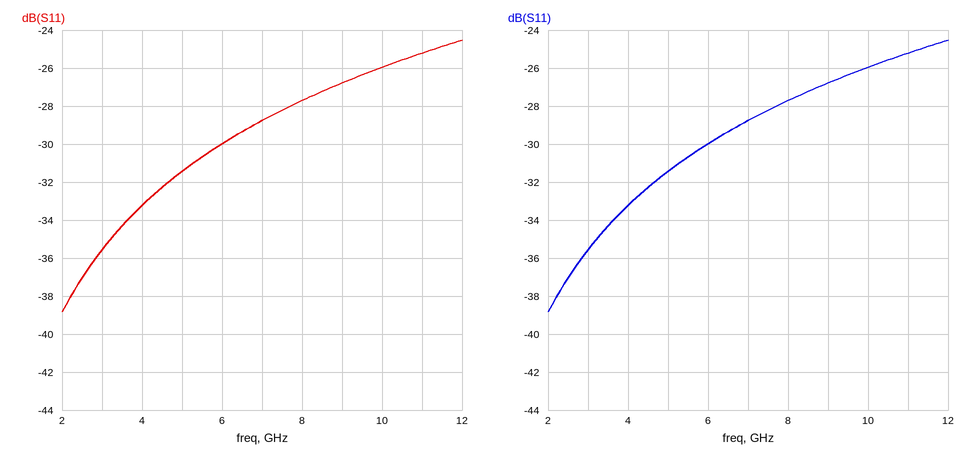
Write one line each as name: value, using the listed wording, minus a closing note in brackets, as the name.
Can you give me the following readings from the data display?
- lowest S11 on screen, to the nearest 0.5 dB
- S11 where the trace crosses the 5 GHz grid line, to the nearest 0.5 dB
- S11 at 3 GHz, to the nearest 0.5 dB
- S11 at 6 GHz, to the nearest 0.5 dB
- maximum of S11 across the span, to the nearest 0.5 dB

lowest S11 on screen, to the nearest 0.5 dB: -39.0 dB
S11 where the trace crosses the 5 GHz grid line, to the nearest 0.5 dB: -31.5 dB
S11 at 3 GHz, to the nearest 0.5 dB: -35.5 dB
S11 at 6 GHz, to the nearest 0.5 dB: -30.0 dB
maximum of S11 across the span, to the nearest 0.5 dB: -24.5 dB
